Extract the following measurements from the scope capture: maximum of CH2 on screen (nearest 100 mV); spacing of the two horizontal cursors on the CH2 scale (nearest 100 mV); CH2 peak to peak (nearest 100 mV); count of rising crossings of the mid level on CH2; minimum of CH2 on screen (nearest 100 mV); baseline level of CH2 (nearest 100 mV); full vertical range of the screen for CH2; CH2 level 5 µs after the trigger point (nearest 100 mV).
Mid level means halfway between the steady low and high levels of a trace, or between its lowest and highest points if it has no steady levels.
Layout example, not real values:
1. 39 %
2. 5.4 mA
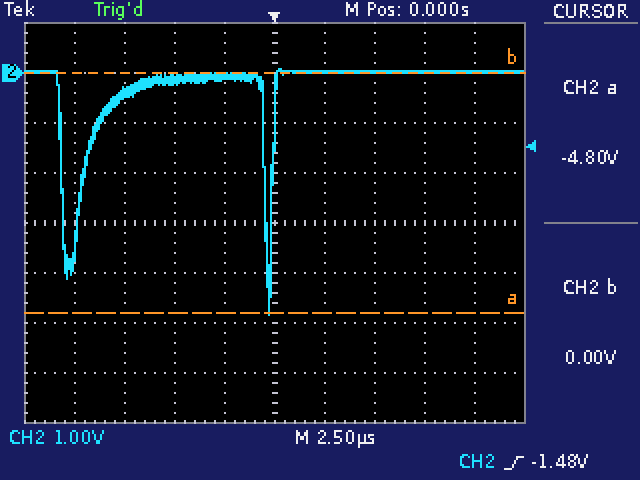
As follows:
1. 100 mV
2. 4.8 V
3. 4.9 V
4. 2
5. -4.8 V
6. 0.0 V
7. 8 V
8. 0.0 V
